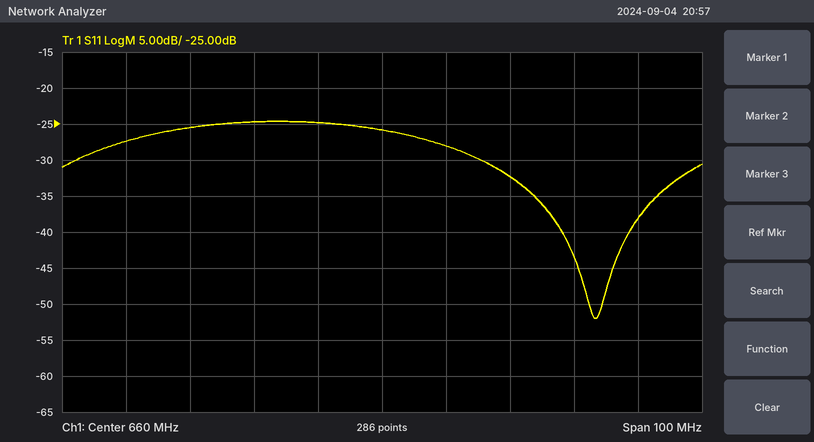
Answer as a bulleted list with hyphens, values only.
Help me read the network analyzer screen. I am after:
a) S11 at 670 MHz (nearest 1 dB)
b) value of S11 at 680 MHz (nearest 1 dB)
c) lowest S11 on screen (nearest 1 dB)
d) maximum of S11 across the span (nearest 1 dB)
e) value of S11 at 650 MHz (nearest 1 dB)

- -28 dB
- -32 dB
- -52 dB
- -25 dB
- -25 dB
